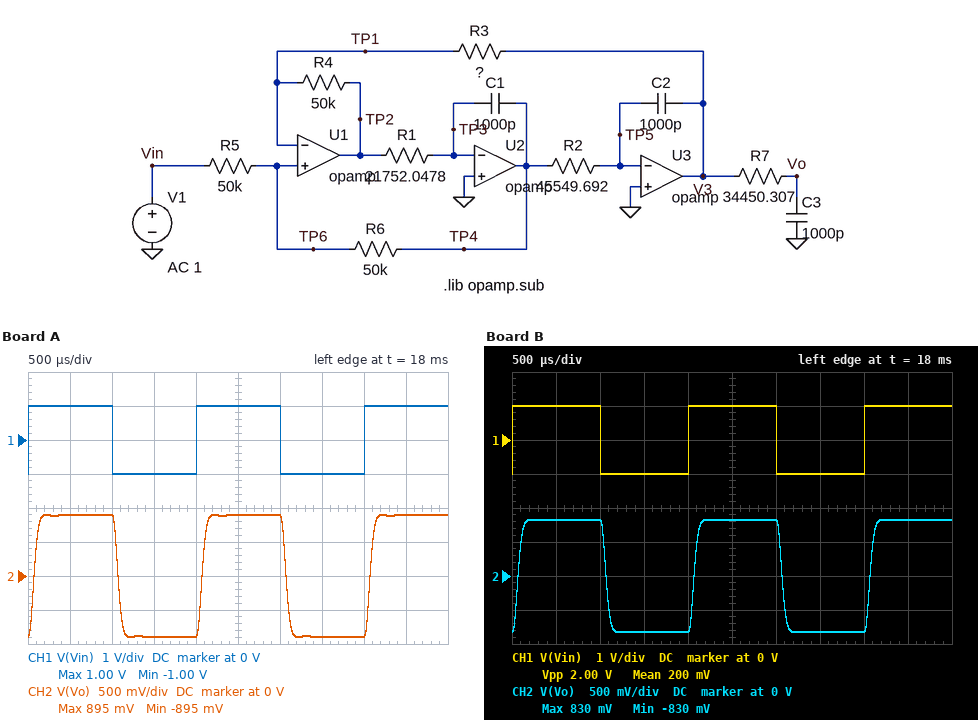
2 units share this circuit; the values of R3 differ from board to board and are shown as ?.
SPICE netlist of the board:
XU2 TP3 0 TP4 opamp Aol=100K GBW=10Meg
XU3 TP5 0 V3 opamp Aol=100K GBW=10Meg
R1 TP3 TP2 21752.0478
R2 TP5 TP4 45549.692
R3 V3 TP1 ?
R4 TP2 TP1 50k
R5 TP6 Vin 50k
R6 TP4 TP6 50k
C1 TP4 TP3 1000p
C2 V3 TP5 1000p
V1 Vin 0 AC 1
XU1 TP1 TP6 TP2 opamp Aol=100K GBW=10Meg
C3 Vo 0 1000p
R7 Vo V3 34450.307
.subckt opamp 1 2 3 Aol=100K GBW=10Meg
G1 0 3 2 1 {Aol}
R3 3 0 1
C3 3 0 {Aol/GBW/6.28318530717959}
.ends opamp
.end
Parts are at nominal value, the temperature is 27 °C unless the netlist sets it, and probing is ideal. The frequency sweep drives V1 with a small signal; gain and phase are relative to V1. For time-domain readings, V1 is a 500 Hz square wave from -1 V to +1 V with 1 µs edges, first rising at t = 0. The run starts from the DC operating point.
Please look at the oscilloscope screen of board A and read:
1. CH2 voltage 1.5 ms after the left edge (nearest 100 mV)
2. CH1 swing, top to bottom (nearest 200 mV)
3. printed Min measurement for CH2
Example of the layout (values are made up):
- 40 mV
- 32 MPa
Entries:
- -900 mV
- 2.0 V
- -895 mV
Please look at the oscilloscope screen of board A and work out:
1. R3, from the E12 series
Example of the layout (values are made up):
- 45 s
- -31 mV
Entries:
- 39 kΩ
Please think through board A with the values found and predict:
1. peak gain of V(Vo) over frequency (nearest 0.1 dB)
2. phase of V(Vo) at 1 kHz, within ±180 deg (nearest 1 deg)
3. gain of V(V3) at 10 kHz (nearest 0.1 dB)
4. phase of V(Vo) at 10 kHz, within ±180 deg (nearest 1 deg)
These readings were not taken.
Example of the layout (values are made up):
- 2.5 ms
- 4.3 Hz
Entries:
- -1.0 dB
- -27 deg
- -11.3 dB
- 166 deg
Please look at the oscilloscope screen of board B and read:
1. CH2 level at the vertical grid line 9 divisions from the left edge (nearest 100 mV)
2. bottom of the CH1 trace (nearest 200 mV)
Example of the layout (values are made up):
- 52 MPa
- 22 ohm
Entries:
- 800 mV
- -1.0 V
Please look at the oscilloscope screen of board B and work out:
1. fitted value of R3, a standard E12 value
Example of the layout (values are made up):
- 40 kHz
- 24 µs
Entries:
- 33 kΩ
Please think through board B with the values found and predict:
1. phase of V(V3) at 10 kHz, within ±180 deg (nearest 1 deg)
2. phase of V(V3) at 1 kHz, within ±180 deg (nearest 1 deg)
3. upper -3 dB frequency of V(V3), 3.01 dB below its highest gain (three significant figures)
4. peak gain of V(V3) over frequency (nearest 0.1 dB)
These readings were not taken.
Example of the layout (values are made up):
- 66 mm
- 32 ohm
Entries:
- -124 deg
- -14 deg
- 5.95 kHz
- -1.6 dB
